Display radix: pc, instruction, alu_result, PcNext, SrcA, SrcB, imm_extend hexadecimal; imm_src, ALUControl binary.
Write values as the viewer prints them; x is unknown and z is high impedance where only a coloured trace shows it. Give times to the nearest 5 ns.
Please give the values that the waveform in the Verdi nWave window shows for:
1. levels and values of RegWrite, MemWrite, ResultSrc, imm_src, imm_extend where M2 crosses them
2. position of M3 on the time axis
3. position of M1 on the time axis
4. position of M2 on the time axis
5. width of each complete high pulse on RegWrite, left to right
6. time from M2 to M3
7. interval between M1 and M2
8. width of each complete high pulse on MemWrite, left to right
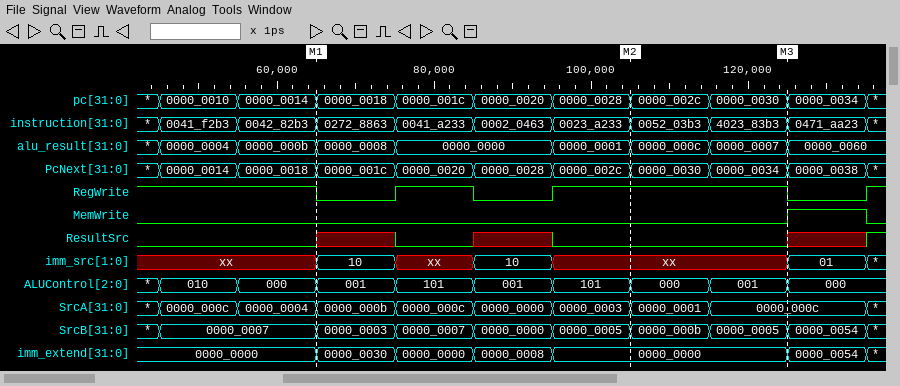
RegWrite=1, MemWrite=0, ResultSrc=0, imm_src=xx, imm_extend=0000_0000
125 ns
65 ns
105 ns
10 ns, 30 ns
20 ns
40 ns
10 ns
